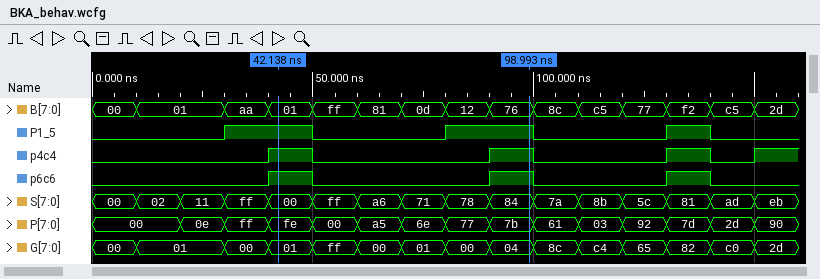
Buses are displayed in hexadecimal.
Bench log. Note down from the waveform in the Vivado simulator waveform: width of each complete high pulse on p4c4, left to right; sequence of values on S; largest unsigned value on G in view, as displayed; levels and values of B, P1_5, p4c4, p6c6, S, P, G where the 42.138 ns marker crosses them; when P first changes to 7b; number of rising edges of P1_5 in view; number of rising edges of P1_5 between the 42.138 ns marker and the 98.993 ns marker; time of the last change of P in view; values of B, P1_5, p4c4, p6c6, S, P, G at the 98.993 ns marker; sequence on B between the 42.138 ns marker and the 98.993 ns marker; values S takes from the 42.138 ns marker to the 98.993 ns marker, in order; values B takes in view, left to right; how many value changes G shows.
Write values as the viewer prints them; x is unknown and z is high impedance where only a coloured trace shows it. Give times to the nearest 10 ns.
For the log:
10 ns, 10 ns, 10 ns
00, 02, 11, ff, 00, ff, a6, 71, 78, 84, 7a, 8b, 5c, 81, ad, eb
ff
B=01, P1_5=1, p4c4=1, p6c6=1, S=00, P=fe, G=01
90 ns
3
1
150 ns
B=76, P1_5=1, p4c4=1, p6c6=1, S=84, P=7b, G=04
01, ff, 81, 0d, 12, 76
00, ff, a6, 71, 78, 84
00, 01, aa, 01, ff, 81, 0d, 12, 76, 8c, c5, 77, f2, c5, 2d
14
